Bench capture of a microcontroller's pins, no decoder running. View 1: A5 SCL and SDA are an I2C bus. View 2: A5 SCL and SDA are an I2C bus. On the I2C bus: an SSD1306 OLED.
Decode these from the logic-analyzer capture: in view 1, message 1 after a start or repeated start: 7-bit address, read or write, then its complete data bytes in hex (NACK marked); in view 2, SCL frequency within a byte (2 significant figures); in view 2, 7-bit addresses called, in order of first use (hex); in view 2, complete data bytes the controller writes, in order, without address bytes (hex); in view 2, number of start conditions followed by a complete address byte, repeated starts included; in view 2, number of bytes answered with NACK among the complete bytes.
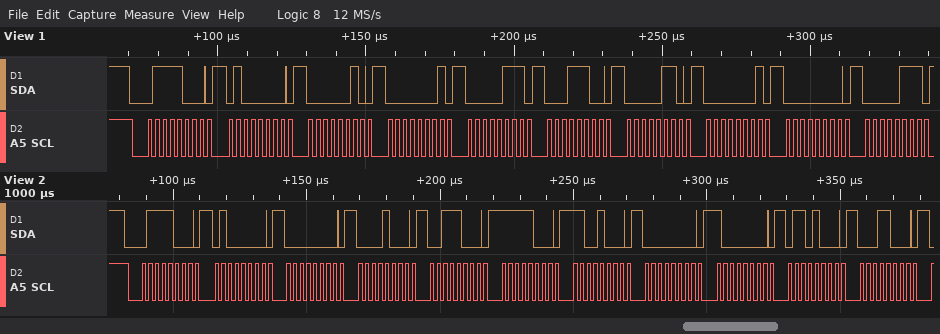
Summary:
0x3C write: 40 02 01 07 1C 06 01 00 07
400 kHz
0x3C
40 00 08 38 F8 C8 00 80 68 18
1
0
